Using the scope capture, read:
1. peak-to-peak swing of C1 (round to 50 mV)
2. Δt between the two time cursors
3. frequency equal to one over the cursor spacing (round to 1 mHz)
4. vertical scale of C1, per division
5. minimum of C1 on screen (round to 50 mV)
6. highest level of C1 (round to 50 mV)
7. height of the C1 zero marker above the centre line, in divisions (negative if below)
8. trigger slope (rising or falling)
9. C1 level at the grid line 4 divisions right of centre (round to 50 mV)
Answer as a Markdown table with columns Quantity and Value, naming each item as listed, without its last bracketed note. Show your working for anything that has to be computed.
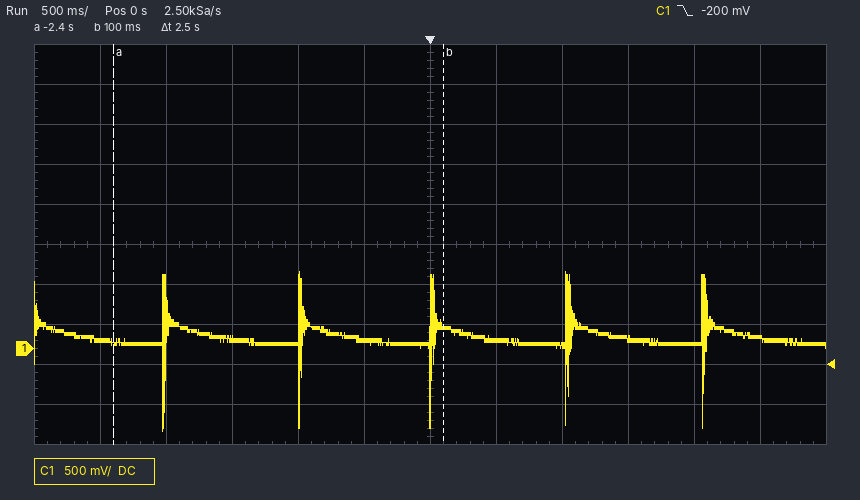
| Quantity | Value |
|---|---|
| peak-to-peak swing of C1 | 950 mV − (-1.05 V) = 2.00 V |
| Δt between the two time cursors | 2.5 s |
| frequency equal to one over the cursor spacing | 1 / 2.5 s ≈ 400 mHz |
| vertical scale of C1, per division | 500 mV |
| minimum of C1 on screen | -1.05 V |
| highest level of C1 | 950 mV |
| height of the C1 zero marker above the centre line, in divisions | -2.6 div |
| trigger slope | falling |
| C1 level at the grid line 4 divisions right of centre | 50 mV |
